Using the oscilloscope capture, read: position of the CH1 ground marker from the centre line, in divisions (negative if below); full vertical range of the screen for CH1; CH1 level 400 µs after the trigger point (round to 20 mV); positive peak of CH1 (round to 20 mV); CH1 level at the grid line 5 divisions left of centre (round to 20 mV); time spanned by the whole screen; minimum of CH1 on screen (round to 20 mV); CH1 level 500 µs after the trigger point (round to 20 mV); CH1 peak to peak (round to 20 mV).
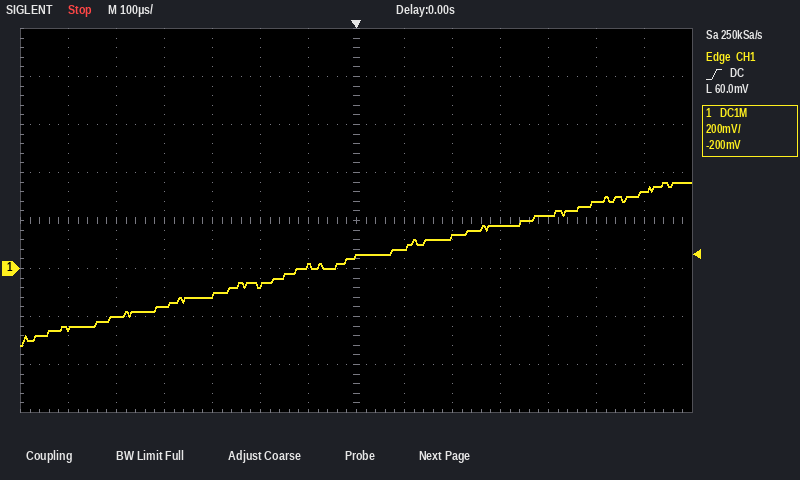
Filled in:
-1.0 div
1.6 V
220 mV
360 mV
-200 mV
1.4 ms
-320 mV
280 mV
680 mV
